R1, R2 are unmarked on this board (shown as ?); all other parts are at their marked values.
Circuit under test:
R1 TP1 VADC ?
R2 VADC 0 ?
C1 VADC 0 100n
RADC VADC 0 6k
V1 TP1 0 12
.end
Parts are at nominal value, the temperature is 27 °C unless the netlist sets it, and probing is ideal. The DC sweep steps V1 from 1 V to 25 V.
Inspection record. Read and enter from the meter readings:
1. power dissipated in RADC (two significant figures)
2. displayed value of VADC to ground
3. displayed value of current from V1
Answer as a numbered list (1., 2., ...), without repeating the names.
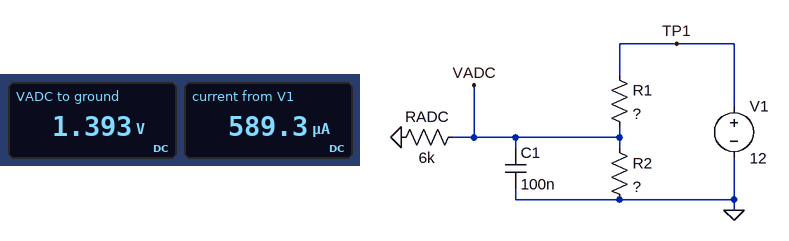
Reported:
1. 320 µW
2. 1.393 V
3. 589.3 µA
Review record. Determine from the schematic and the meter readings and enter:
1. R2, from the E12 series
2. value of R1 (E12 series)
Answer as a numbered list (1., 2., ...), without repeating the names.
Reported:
1. 3.9 kΩ
2. 18 kΩ
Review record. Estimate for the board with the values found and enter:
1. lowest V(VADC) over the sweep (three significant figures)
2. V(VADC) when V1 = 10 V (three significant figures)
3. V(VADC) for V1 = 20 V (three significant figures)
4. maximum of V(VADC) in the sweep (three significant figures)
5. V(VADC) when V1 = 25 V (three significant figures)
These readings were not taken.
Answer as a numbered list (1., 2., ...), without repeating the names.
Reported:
1. 116 mV
2. 1.16 V
3. 2.32 V
4. 2.90 V
5. 2.90 V
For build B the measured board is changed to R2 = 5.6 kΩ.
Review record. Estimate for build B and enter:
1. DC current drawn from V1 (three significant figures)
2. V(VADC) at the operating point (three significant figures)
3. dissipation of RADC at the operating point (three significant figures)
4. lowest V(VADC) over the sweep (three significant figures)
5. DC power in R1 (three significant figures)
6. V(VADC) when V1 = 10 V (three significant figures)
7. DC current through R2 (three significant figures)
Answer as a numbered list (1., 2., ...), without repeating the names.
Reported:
1. 574 µA
2. 1.66 V
3. 461 µW
4. 139 mV
5. 5.94 mW
6. 1.39 V
7. 297 µA
